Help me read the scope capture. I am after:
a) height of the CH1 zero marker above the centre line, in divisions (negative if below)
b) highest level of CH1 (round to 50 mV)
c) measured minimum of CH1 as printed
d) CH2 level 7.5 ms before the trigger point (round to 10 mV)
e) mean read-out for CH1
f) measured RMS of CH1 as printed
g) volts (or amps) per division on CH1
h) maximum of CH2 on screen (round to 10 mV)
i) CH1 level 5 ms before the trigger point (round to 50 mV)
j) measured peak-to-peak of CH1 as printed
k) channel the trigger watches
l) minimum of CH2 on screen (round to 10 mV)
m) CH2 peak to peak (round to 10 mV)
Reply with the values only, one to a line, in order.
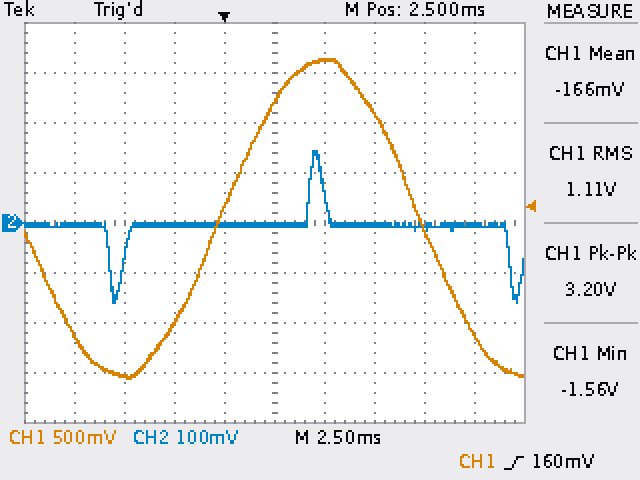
0.0 div
1.65 V
-1.56 V
0 mV
-166 mV
1.11 V
500 mV
140 mV
-1.55 V
3.20 V
CH1
-160 mV
300 mV
